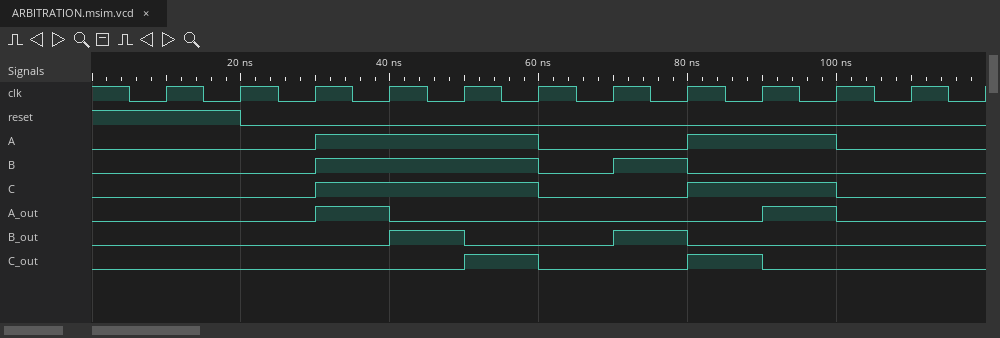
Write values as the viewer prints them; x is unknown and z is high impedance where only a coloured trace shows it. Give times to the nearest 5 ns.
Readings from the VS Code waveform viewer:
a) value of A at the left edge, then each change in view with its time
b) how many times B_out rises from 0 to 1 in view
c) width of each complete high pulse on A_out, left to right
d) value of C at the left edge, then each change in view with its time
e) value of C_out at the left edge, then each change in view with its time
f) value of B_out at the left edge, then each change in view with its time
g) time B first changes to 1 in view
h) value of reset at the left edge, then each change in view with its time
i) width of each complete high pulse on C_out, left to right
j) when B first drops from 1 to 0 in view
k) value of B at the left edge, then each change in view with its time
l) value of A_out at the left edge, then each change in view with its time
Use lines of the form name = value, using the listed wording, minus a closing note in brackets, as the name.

value of A at the left edge, then each change in view with its time = 0, 1 at 30 ns, 0 at 60 ns, 1 at 80 ns, 0 at 100 ns
how many times B_out rises from 0 to 1 in view = 2
width of each complete high pulse on A_out, left to right = 10 ns, 10 ns
value of C at the left edge, then each change in view with its time = 0, 1 at 30 ns, 0 at 60 ns, 1 at 80 ns, 0 at 100 ns
value of C_out at the left edge, then each change in view with its time = 0, 1 at 50 ns, 0 at 60 ns, 1 at 80 ns, 0 at 90 ns
value of B_out at the left edge, then each change in view with its time = 0, 1 at 40 ns, 0 at 50 ns, 1 at 70 ns, 0 at 80 ns
time B first changes to 1 in view = 30 ns
value of reset at the left edge, then each change in view with its time = 1, 0 at 20 ns
width of each complete high pulse on C_out, left to right = 10 ns, 10 ns
when B first drops from 1 to 0 in view = 60 ns
value of B at the left edge, then each change in view with its time = 0, 1 at 30 ns, 0 at 60 ns, 1 at 70 ns, 0 at 80 ns
value of A_out at the left edge, then each change in view with its time = 0, 1 at 30 ns, 0 at 40 ns, 1 at 90 ns, 0 at 100 ns
